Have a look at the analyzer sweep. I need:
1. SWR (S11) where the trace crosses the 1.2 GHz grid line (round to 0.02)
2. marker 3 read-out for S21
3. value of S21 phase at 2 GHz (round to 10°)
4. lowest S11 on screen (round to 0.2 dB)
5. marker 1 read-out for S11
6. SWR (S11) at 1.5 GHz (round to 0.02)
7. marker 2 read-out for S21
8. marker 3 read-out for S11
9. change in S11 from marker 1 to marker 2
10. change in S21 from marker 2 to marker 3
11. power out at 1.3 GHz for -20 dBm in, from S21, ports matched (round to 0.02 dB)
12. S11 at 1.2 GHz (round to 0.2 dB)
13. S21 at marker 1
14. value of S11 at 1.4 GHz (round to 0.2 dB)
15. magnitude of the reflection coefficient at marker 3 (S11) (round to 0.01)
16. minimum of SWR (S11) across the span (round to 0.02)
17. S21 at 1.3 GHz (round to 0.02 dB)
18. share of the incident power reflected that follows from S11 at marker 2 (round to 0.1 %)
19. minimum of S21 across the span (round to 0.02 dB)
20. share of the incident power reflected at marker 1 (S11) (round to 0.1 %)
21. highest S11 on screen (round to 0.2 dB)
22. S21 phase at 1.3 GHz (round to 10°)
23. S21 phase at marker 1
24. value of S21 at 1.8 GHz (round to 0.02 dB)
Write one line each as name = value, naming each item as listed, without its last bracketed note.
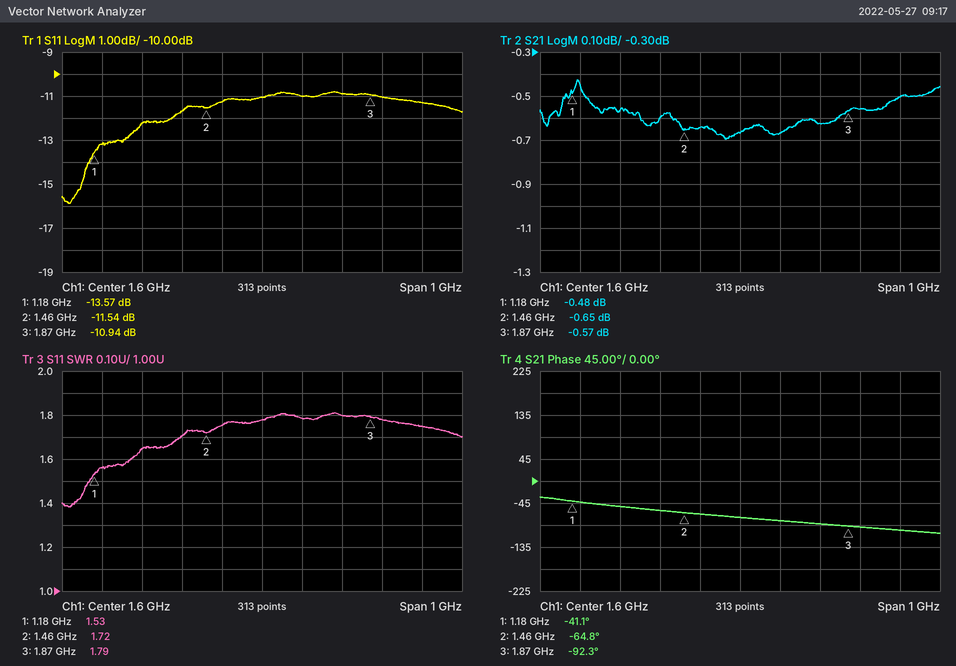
SWR (S11) where the trace crosses the 1.2 GHz grid line = 1.56
marker 3 read-out for S21 = -0.57 dB
value of S21 phase at 2 GHz = -100°
lowest S11 on screen = -15.8 dB
marker 1 read-out for S11 = -13.57 dB
SWR (S11) at 1.5 GHz = 1.76
marker 2 read-out for S21 = -0.65 dB
marker 3 read-out for S11 = -10.94 dB
change in S11 from marker 1 to marker 2 = 2.03 dB
change in S21 from marker 2 to marker 3 = 0.08 dB
power out at 1.3 GHz for -20 dBm in, from S21, ports matched = -20.56 dBm
S11 at 1.2 GHz = -13.2 dB
S21 at marker 1 = -0.48 dB
value of S11 at 1.4 GHz = -11.6 dB
magnitude of the reflection coefficient at marker 3 (S11) = 0.28
minimum of SWR (S11) across the span = 1.38
S21 at 1.3 GHz = -0.56 dB
share of the incident power reflected that follows from S11 at marker 2 = 7.0 %
minimum of S21 across the span = -0.70 dB
share of the incident power reflected at marker 1 (S11) = 4.4 %
highest S11 on screen = -10.8 dB
S21 phase at 1.3 GHz = -50°
S21 phase at marker 1 = -41.1°
value of S21 at 1.8 GHz = -0.62 dB
